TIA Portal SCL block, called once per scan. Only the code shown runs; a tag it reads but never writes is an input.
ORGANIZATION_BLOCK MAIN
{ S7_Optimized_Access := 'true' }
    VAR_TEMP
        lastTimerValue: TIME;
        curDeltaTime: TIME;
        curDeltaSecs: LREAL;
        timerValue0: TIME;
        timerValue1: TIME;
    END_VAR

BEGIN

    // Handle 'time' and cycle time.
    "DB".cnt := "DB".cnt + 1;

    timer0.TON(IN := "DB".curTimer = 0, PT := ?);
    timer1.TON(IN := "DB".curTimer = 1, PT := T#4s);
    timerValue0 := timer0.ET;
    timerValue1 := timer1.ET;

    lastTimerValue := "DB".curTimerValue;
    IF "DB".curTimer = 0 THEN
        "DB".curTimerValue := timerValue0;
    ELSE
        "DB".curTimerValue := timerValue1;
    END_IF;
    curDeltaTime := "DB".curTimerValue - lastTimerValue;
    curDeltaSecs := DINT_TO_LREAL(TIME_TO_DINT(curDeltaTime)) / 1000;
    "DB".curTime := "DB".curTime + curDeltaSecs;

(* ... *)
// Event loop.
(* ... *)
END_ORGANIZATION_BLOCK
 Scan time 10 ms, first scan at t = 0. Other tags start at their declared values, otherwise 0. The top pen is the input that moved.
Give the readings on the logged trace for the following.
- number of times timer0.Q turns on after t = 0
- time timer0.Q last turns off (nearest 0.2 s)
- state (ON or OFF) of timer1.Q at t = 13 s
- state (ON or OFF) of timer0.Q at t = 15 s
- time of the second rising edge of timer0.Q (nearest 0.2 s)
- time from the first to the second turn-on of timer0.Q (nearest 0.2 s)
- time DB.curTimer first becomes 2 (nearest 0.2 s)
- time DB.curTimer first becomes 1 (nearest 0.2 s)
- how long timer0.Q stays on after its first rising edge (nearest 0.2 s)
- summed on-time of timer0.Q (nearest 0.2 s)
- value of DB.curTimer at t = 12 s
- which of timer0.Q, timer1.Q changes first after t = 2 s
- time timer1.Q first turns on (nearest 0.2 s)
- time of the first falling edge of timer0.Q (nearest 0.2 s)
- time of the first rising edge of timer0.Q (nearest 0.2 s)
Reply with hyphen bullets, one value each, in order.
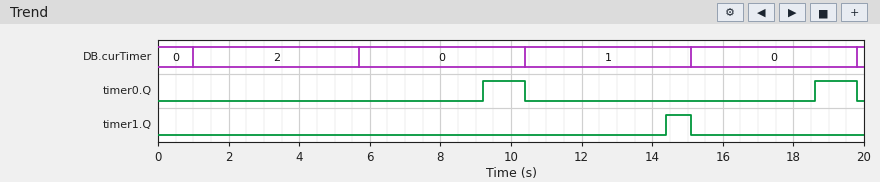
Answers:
- 2
- 19.8 s
- OFF
- OFF
- 18.6 s
- 9.4 s
- 1.0 s
- 10.4 s
- 1.2 s
- 2.4 s
- 1
- timer0.Q
- 14.4 s
- 10.4 s
- 9.2 s
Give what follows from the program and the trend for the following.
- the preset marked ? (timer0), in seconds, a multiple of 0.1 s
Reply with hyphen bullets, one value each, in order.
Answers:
- 3.5 s
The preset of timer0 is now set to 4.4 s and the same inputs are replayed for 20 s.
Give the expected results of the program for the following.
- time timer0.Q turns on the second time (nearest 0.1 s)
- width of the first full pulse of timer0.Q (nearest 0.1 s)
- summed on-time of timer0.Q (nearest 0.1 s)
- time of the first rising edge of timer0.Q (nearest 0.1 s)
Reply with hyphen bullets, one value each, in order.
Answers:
- 19.5 s
- 0.3 s
- 0.6 s
- 10.1 s
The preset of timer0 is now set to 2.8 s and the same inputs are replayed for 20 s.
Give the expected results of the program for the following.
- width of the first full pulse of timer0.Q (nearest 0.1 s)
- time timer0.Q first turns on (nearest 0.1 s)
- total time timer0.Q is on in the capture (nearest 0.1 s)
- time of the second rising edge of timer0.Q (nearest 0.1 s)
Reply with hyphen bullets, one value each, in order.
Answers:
- 1.9 s
- 8.5 s
- 3.8 s
- 17.9 s
